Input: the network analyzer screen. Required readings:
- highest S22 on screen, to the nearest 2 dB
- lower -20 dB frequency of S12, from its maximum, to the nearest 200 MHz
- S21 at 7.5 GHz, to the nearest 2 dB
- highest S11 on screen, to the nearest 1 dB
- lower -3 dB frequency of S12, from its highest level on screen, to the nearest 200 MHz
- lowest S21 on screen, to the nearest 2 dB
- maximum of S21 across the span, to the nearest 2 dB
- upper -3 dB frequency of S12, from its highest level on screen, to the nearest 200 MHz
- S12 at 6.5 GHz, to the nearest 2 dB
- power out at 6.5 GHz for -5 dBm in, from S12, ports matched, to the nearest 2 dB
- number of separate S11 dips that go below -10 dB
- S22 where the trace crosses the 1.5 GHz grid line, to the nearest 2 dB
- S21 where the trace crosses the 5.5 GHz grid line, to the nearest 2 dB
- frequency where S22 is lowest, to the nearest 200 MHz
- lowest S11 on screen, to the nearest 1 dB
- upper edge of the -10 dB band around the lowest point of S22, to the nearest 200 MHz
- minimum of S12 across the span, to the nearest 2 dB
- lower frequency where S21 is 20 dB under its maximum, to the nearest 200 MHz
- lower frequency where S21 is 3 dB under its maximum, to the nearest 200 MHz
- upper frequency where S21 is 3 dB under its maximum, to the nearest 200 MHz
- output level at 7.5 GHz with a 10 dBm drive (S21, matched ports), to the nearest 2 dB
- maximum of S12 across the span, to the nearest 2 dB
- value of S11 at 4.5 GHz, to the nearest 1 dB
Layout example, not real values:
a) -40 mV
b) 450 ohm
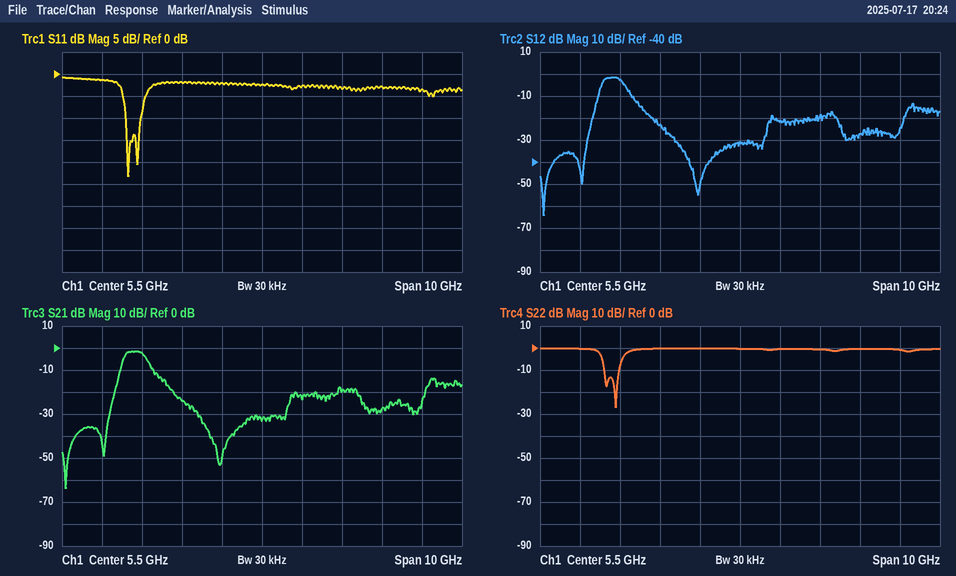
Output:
a) 0 dB
b) 1.8 GHz
c) -20 dB
d) -1 dB
e) 2.0 GHz
f) -64 dB
g) -2 dB
h) 2.6 GHz
i) -22 dB
j) -26 dBm
k) 2
l) 0 dB
m) -32 dB
n) 2.4 GHz
o) -23 dB
p) 2.4 GHz
q) -64 dB
r) 1.8 GHz
s) 2.0 GHz
t) 2.6 GHz
u) -10 dBm
v) -2 dB
w) -2 dB
